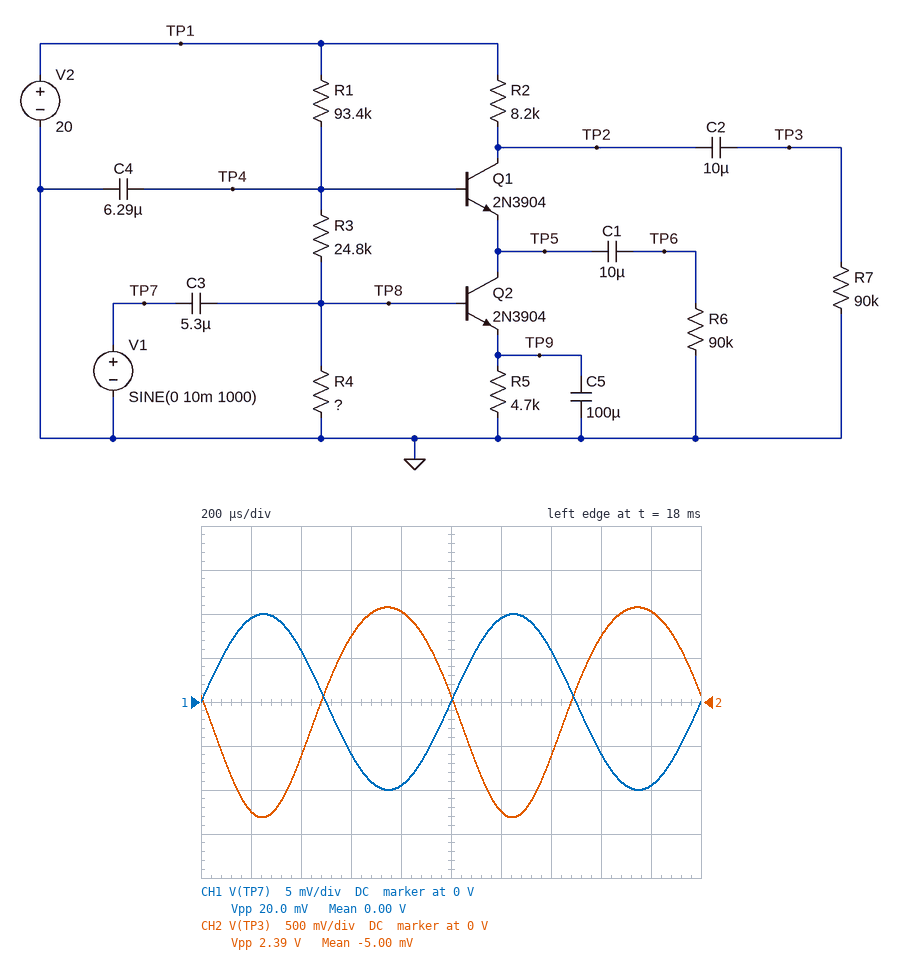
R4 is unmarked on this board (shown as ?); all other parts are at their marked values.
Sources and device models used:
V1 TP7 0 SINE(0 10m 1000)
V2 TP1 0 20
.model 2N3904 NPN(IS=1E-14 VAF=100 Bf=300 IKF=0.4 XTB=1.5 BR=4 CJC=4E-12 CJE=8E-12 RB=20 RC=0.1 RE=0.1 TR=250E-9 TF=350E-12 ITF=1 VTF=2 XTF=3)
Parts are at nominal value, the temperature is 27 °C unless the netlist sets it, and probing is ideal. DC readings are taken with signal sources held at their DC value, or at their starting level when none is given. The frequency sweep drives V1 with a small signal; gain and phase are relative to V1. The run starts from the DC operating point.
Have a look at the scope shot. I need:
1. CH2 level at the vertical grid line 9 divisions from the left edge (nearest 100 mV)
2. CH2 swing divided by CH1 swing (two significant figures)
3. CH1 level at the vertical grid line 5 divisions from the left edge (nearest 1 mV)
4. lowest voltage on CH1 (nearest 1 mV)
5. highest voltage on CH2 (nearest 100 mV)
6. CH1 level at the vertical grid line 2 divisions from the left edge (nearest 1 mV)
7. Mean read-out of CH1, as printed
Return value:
1.0 V
120
0 V
-10 mV
1.1 V
6 mV
0.00 V
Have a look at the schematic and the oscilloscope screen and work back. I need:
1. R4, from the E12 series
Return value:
18 kΩ
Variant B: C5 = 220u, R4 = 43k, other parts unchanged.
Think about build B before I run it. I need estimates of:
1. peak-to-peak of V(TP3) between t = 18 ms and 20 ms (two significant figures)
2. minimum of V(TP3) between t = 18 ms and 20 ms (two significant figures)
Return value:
5.4 V
-3.0 V
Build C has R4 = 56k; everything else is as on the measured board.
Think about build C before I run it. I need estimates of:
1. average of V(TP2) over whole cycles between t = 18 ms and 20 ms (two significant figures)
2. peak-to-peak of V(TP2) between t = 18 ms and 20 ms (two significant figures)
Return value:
11 V
5.4 V
